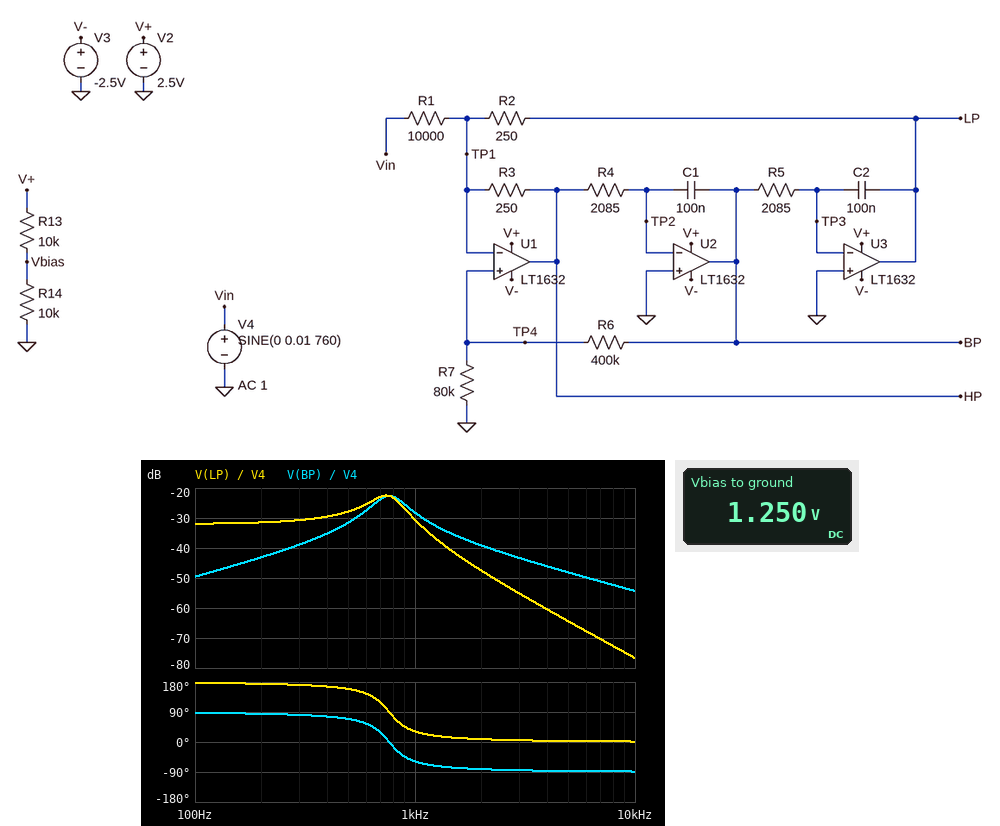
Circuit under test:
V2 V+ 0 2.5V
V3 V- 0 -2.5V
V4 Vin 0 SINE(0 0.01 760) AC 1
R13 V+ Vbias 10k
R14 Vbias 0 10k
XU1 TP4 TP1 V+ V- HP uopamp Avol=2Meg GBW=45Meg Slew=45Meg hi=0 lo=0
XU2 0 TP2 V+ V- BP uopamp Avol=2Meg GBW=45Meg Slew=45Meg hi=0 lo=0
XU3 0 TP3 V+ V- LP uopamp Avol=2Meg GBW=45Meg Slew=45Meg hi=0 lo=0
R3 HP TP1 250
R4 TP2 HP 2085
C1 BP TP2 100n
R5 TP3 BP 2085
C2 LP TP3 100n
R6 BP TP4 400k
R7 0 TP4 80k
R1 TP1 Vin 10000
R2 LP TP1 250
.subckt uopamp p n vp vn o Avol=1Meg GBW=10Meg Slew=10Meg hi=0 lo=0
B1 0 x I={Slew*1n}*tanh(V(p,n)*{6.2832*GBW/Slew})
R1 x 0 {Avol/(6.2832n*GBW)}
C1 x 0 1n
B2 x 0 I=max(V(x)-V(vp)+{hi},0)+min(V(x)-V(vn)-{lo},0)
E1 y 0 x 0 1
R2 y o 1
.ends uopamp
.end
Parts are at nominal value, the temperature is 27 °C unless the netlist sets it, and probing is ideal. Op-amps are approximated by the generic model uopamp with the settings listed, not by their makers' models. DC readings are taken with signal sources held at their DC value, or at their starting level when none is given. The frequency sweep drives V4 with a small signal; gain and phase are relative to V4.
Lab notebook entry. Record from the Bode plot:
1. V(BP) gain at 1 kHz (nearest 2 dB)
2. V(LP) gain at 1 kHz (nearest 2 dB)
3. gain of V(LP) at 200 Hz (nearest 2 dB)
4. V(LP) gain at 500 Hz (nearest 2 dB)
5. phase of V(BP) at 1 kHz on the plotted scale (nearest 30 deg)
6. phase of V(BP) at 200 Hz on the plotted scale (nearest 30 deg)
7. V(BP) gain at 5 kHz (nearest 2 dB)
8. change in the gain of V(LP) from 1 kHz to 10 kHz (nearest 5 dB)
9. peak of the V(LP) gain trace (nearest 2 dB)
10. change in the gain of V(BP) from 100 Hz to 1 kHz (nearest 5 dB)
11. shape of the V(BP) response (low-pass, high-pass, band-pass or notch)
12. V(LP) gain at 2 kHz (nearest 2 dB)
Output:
-28 dB
-30 dB
-32 dB
-28 dB
-60 deg
90 deg
-48 dB
-45 dB
-22 dB
20 dB
band-pass
-48 dB
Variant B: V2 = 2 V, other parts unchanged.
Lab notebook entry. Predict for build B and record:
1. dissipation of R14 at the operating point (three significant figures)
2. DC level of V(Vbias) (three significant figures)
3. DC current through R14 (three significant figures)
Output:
100 µW
1.00 V
100 µA
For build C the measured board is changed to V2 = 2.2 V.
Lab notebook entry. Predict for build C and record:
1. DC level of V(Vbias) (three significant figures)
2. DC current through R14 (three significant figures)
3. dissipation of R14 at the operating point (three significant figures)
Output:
1.10 V
110 µA
121 µW
